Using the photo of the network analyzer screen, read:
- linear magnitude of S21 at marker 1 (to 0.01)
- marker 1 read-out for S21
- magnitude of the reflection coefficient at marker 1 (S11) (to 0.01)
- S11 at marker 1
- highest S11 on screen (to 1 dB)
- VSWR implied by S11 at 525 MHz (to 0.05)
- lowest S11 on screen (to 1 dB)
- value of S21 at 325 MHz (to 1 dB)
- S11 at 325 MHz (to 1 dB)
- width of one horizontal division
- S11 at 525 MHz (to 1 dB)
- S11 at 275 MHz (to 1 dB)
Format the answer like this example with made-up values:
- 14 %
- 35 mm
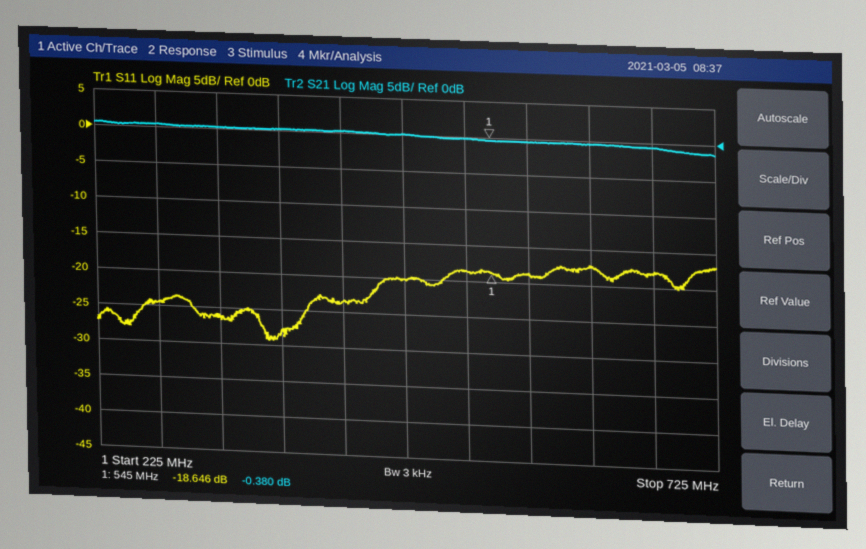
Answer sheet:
- 0.96
- -0.380 dB
- 0.12
- -18.646 dB
- -17 dB
- 1.25
- -29 dB
- 0 dB
- -26 dB
- 50 MHz
- -19 dB
- -25 dB
